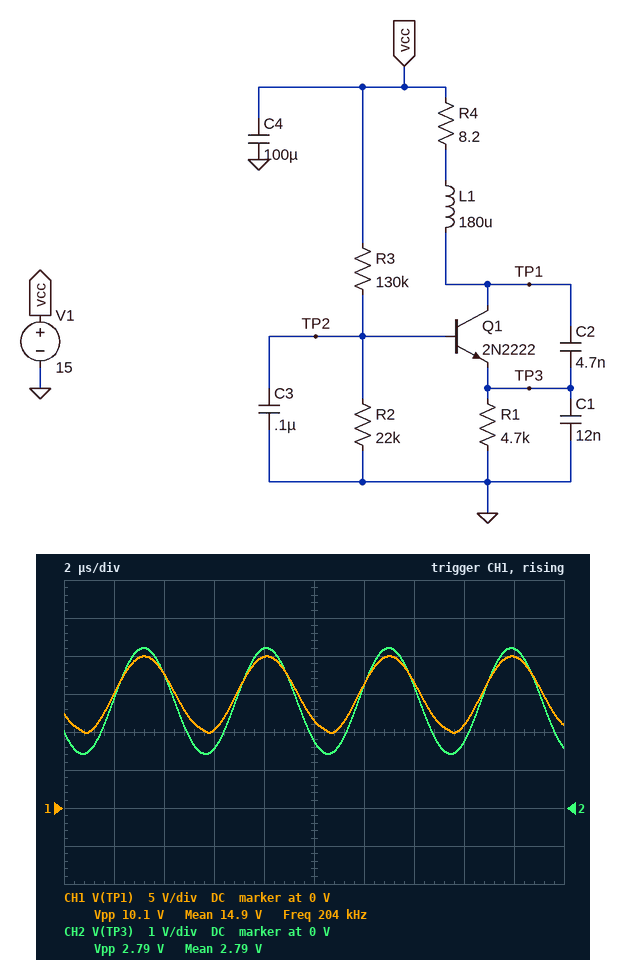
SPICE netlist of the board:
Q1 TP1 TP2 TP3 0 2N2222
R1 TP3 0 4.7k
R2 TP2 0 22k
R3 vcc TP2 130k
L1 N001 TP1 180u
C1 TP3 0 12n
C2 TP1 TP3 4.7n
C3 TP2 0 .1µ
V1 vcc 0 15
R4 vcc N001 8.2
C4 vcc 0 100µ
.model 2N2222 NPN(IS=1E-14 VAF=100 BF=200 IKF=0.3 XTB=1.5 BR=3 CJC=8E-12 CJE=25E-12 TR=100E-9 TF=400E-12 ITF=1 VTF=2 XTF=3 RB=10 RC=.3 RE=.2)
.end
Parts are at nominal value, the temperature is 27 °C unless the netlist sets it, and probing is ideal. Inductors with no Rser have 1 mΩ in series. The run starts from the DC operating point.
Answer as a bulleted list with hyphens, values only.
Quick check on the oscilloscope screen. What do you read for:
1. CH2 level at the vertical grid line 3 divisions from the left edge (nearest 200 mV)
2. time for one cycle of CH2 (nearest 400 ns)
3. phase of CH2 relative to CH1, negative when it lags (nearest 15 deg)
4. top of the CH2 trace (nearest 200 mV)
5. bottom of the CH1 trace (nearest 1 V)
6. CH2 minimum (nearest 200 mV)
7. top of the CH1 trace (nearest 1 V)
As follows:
- 1.6 V
- 4.8 µs
- 0 deg
- 4.2 V
- 10 V
- 1.4 V
- 20 V
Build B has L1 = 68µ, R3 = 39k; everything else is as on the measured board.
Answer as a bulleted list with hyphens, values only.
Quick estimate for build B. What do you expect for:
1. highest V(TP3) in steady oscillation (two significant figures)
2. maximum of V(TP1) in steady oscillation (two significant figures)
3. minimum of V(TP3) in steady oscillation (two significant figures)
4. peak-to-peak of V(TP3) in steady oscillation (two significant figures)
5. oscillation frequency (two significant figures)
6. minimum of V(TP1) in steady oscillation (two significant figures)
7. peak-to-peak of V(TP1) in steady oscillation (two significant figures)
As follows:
- 6.9 V
- 19 V
- 4.6 V
- 2.3 V
- 330 kHz
- 11 V
- 8.3 V
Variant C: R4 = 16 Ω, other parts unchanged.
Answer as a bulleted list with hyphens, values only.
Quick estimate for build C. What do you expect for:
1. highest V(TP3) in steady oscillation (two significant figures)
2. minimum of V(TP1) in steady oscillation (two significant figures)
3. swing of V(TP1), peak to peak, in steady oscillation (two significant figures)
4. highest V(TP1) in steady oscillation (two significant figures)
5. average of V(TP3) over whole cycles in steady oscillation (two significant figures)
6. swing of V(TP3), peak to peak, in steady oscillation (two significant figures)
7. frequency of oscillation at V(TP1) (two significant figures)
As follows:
- 2.5 V
- 13 V
- 3.8 V
- 17 V
- 2.0 V
- 1.0 V
- 200 kHz
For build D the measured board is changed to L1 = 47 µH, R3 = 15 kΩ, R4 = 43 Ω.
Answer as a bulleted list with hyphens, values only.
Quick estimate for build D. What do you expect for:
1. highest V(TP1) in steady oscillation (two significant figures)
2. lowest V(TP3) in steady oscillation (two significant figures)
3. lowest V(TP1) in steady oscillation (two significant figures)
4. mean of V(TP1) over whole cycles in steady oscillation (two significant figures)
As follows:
- 16 V
- 8.1 V
- 13 V
- 15 V
